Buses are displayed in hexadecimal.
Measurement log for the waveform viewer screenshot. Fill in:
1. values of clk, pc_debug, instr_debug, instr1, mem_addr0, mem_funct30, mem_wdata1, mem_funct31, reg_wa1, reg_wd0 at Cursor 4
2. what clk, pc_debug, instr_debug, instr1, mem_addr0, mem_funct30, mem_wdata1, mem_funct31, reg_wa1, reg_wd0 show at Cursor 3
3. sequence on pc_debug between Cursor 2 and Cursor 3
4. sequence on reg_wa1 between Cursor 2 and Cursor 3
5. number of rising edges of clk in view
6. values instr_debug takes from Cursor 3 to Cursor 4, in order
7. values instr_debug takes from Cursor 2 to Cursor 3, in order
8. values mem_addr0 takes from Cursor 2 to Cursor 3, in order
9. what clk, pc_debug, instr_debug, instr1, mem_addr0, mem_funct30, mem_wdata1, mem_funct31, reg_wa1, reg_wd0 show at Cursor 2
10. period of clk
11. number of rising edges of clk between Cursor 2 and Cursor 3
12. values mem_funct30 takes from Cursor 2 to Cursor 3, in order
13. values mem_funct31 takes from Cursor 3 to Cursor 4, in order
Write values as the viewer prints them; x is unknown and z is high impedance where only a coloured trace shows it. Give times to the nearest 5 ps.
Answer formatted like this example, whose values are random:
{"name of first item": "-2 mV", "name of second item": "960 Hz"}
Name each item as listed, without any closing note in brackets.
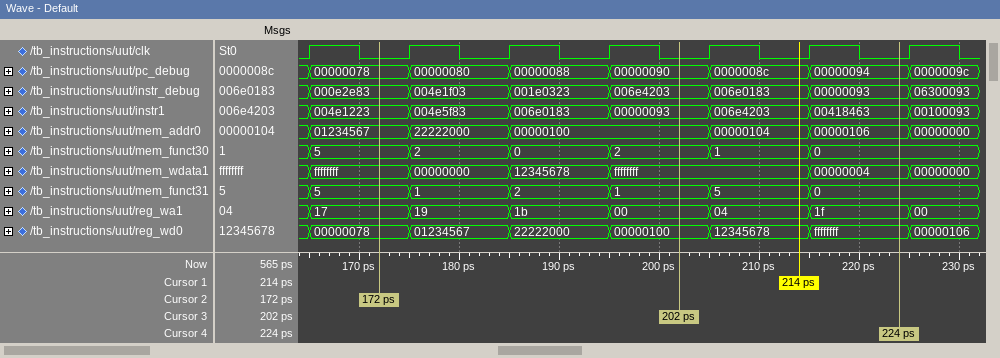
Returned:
{"values of clk, pc_debug, instr_debug, instr1, mem_addr0, mem_funct30, mem_wdata1, mem_funct31, reg_wa1, reg_wd0 at Cursor 4": "clk=0, pc_debug=00000094, instr_debug=00000093, instr1=00418463, mem_addr0=00000106, mem_funct30=0, mem_wdata1=00000004, mem_funct31=0, reg_wa1=1f, reg_wd0=ffffffff", "what clk, pc_debug, instr_debug, instr1, mem_addr0, mem_funct30, mem_wdata1, mem_funct31, reg_wa1, reg_wd0 show at Cursor 3": "clk=0, pc_debug=00000090, instr_debug=006e4203, instr1=00000093, mem_addr0=00000100, mem_funct30=2, mem_wdata1=ffffffff, mem_funct31=1, reg_wa1=00, reg_wd0=00000100", "sequence on pc_debug between Cursor 2 and Cursor 3": "00000078, 00000080, 00000088, 00000090", "sequence on reg_wa1 between Cursor 2 and Cursor 3": "17, 19, 1b, 00", "number of rising edges of clk in view": "7", "values instr_debug takes from Cursor 3 to Cursor 4, in order": "006e4203, 006e0183, 00000093", "values instr_debug takes from Cursor 2 to Cursor 3, in order": "000e2e83, 004e1f03, 001e0323, 006e4203", "values mem_addr0 takes from Cursor 2 to Cursor 3, in order": "01234567, 22222000, 00000100", "what clk, pc_debug, instr_debug, instr1, mem_addr0, mem_funct30, mem_wdata1, mem_funct31, reg_wa1, reg_wd0 show at Cursor 2": "clk=0, pc_debug=00000078, instr_debug=000e2e83, instr1=004e1223, mem_addr0=01234567, mem_funct30=5, mem_wdata1=ffffffff, mem_funct31=5, reg_wa1=17, reg_wd0=00000078", "period of clk": "10 ps", "number of rising edges of clk between Cursor 2 and Cursor 3": "3", "values mem_funct30 takes from Cursor 2 to Cursor 3, in order": "5, 2, 0, 2", "values mem_funct31 takes from Cursor 3 to Cursor 4, in order": "1, 5, 0"}
